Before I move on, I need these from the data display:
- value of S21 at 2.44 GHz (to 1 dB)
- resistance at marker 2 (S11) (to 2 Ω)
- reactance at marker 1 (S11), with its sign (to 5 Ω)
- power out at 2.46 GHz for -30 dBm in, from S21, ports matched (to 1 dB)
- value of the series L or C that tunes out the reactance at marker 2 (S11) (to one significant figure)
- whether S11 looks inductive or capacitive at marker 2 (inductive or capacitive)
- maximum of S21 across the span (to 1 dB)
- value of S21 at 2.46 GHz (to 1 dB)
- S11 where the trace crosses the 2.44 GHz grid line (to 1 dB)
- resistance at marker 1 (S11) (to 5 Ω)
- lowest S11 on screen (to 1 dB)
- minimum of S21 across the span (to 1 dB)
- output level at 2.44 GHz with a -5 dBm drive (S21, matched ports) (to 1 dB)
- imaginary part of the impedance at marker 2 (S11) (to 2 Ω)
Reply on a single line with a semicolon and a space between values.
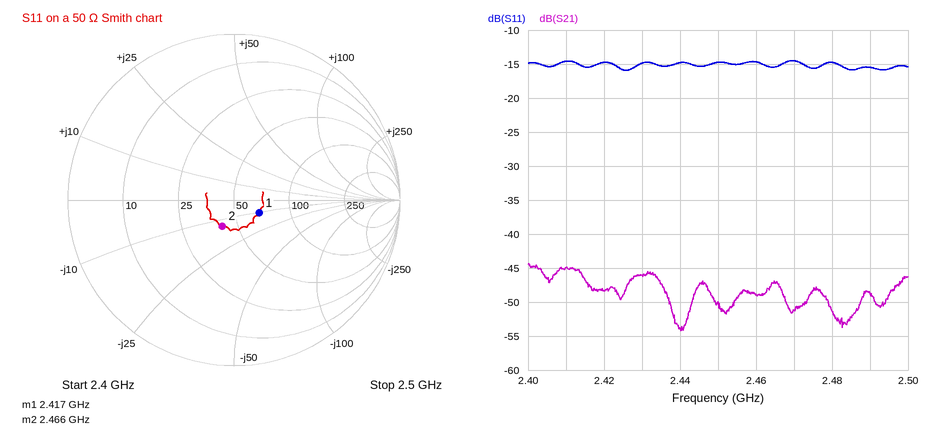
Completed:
-54 dB; 42 Ω; -10 Ω; -79 dBm; 900 pH; capacitive; -44 dB; -49 dB; -15 dB; 65 Ω; -16 dB; -54 dB; -59 dBm; -14 Ω
